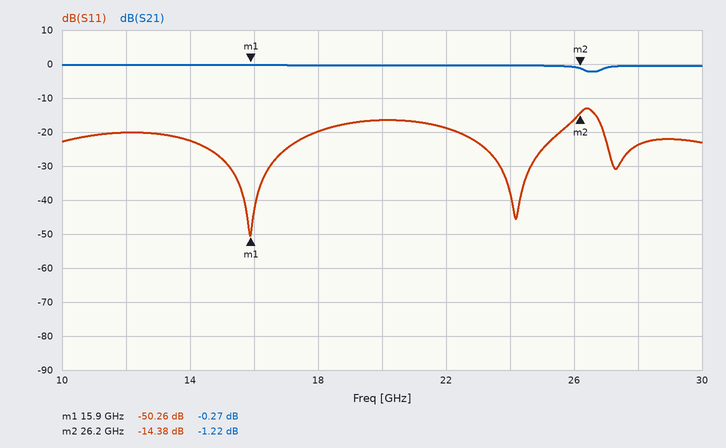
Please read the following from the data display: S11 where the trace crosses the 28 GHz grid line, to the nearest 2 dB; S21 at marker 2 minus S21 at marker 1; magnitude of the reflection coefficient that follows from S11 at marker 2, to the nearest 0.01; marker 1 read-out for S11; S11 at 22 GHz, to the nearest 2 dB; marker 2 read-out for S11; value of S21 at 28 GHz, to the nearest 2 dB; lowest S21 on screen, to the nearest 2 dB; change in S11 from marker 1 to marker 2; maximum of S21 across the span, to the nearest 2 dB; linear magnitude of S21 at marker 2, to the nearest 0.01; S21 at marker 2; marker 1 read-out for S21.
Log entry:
-24 dB
-0.95 dB
0.19
-50.26 dB
-18 dB
-14.38 dB
0 dB
-2 dB
35.88 dB
0 dB
0.87
-1.22 dB
-0.27 dB
